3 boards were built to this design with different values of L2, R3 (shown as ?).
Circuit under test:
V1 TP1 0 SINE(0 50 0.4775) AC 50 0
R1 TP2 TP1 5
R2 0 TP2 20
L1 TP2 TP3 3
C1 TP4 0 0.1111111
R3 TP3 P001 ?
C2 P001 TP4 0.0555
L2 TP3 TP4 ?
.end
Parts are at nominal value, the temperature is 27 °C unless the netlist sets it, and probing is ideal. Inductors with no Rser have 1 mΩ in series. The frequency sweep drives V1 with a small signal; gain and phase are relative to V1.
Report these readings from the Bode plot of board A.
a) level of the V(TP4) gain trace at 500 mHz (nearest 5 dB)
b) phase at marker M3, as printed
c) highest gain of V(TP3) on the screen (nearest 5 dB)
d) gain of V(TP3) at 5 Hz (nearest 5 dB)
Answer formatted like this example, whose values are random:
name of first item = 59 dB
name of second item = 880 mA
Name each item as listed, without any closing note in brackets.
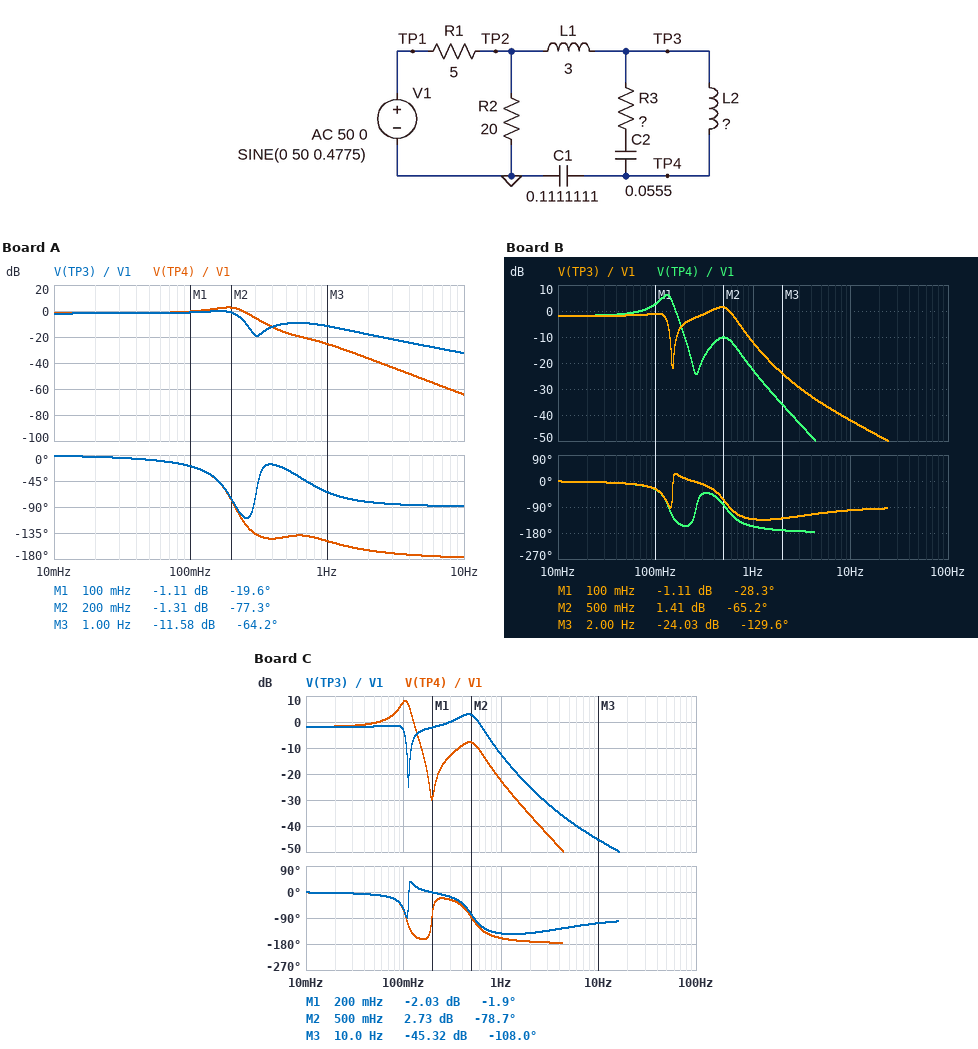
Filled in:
level of the V(TP4) gain trace at 500 mHz = -15 dB
phase at marker M3, as printed = -64.2 deg
highest gain of V(TP3) on the screen = 0 dB
gain of V(TP3) at 5 Hz = -25 dB
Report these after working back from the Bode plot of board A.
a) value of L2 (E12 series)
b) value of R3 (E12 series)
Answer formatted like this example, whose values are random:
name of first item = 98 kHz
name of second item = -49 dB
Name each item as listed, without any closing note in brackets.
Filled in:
value of L2 = 1.8 H
value of R3 = 5.6 Ω
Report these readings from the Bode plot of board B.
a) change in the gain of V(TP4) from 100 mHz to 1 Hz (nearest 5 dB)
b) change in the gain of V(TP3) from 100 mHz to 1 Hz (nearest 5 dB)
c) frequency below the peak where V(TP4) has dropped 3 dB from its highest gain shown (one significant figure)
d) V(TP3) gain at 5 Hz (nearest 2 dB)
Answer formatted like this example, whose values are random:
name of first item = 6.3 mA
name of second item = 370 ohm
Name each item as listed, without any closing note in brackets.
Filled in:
change in the gain of V(TP4) from 100 mHz to 1 Hz = -25 dB
change in the gain of V(TP3) from 100 mHz to 1 Hz = -10 dB
frequency below the peak where V(TP4) has dropped 3 dB from its highest gain shown = 100 mHz
V(TP3) gain at 5 Hz = -36 dB
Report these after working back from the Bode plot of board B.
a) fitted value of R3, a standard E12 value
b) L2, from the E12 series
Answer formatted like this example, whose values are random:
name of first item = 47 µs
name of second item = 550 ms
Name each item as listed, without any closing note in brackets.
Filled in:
fitted value of R3, a standard E12 value = 1.8 Ω
L2, from the E12 series = 6.8 H
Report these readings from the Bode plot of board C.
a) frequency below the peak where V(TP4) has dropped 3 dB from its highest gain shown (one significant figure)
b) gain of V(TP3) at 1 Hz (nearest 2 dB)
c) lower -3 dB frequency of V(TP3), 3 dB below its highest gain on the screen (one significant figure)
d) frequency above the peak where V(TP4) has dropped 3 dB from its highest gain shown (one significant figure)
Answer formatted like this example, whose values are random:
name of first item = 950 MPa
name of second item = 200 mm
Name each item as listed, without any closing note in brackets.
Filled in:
frequency below the peak where V(TP4) has dropped 3 dB from its highest gain shown = 90 mHz
gain of V(TP3) at 1 Hz = -12 dB
lower -3 dB frequency of V(TP3), 3 dB below its highest gain on the screen = 300 mHz
frequency above the peak where V(TP4) has dropped 3 dB from its highest gain shown = 100 mHz
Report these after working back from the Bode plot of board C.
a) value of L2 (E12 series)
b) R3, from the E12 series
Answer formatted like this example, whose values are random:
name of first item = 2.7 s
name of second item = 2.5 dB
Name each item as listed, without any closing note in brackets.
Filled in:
value of L2 = 12 H
R3, from the E12 series = 1.2 Ω
